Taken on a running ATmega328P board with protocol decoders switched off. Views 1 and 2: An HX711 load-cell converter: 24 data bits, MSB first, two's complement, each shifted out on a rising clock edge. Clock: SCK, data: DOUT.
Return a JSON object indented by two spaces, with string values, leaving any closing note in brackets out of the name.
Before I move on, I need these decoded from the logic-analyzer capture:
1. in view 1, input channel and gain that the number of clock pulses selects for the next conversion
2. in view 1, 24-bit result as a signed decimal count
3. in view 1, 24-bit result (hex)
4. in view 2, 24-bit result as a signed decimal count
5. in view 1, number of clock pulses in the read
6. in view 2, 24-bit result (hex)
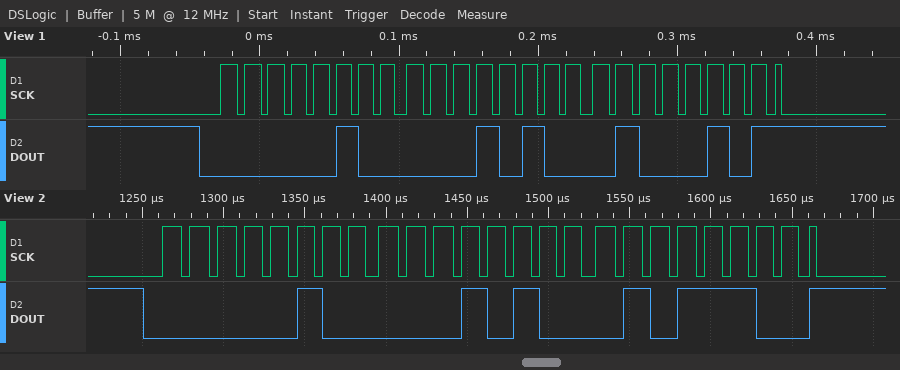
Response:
{
  "in view 1, input channel and gain that the number of clock pulses selects for the next conversion": "channel A, gain 128",
  "in view 1, 24-bit result as a signed decimal count": "267333",
  "in view 1, 24-bit result": "0x041445",
  "in view 2, 24-bit result as a signed decimal count": "267356",
  "in view 1, number of clock pulses in the read": "25",
  "in view 2, 24-bit result": "0x04145C"
}
